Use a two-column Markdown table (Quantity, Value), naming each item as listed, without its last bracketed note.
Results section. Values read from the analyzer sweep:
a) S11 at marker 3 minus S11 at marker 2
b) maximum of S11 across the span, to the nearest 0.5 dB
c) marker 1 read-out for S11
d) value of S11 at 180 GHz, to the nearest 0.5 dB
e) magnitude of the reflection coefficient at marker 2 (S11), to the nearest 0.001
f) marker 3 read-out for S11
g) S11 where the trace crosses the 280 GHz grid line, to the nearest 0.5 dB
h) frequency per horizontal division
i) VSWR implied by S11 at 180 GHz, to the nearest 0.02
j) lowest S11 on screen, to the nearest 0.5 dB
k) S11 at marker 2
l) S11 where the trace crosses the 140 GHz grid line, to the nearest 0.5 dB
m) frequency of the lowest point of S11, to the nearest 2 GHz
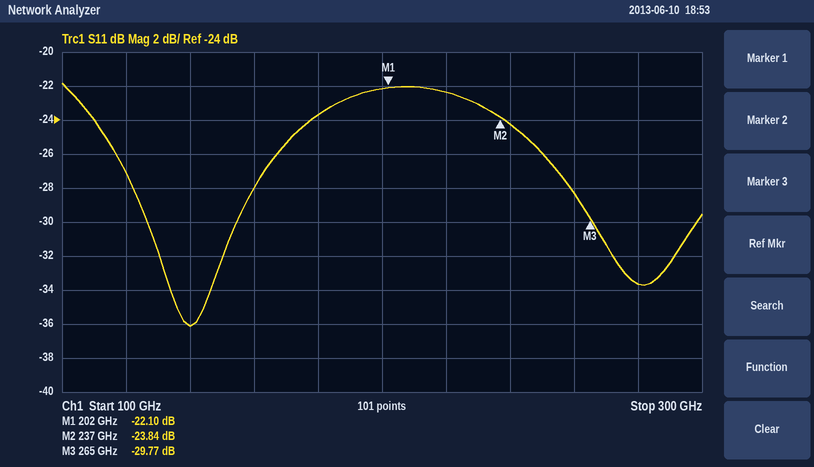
| Quantity | Value |
|---|---|
| S11 at marker 3 minus S11 at marker 2 | -5.93 dB |
| maximum of S11 across the span, to the nearest 0.5 dB | -22.0 dB |
| marker 1 read-out for S11 | -22.10 dB |
| value of S11 at 180 GHz, to the nearest 0.5 dB | -23.5 dB |
| magnitude of the reflection coefficient at marker 2 (S11), to the nearest 0.001 | 0.064 |
| marker 3 read-out for S11 | -29.77 dB |
| S11 where the trace crosses the 280 GHz grid line, to the nearest 0.5 dB | -33.5 dB |
| frequency per horizontal division | 20 GHz |
| VSWR implied by S11 at 180 GHz, to the nearest 0.02 | 1.14 |
| lowest S11 on screen, to the nearest 0.5 dB | -36.0 dB |
| S11 at marker 2 | -23.84 dB |
| S11 where the trace crosses the 140 GHz grid line, to the nearest 0.5 dB | -36.0 dB |
| frequency of the lowest point of S11, to the nearest 2 GHz | 140 GHz |
